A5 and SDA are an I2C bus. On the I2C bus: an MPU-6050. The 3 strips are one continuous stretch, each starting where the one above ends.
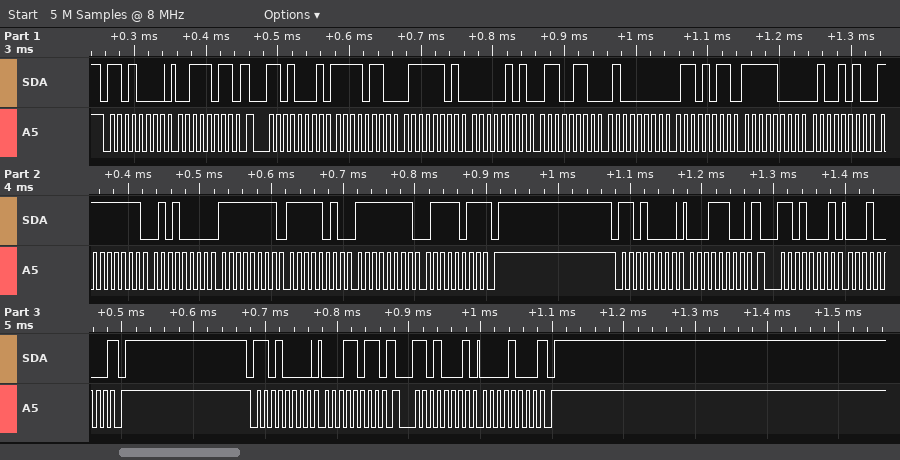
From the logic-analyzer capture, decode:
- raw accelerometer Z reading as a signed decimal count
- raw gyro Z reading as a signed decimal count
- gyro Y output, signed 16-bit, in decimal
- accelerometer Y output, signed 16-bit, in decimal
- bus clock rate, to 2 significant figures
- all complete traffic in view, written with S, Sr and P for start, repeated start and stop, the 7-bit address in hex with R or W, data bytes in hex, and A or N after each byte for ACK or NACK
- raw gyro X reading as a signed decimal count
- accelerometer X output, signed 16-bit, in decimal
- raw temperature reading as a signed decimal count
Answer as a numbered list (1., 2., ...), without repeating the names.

1. 16491
2. -133
3. -6
4. 1382
5. 100 kHz
6. S 68W A 3B A Sr 68R A F6 A 7D A 05 A 66 A 40 A 6B A F8 A 4A A FF A 50 A FF A FA A FF A 7B N P S 68W A 1C A Sr 68R A 10 N P S 68W A 1B A Sr 68R A 08 N P
7. -176
8. -2435
9. -1974
